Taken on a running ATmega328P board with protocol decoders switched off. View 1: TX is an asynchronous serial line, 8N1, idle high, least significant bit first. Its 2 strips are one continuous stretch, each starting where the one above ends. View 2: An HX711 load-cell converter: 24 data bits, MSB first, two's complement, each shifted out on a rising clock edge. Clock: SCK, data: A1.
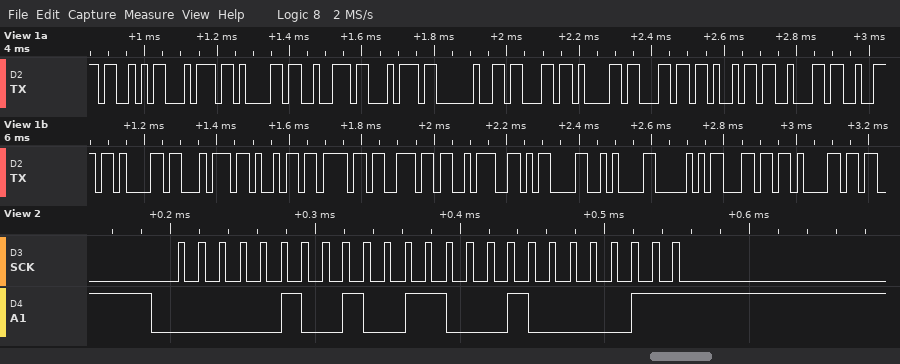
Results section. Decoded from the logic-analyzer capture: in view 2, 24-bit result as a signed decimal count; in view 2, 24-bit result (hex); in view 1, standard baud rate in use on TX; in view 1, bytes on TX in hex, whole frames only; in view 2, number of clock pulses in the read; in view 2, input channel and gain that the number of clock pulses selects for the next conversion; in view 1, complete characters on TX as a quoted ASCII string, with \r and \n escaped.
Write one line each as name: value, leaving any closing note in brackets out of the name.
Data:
in view 2, 24-bit result as a signed decimal count: 301187
in view 2, 24-bit result: 0x049883
in view 1, standard baud rate in use on TX: 57600 baud
in view 1, bytes on TX in hex, whole frames only: 53 74 61 72 74 20 63 61 6C 69 62 72 61 74 69 6F 6E 3A 0D 0A 50 6C 61
in view 2, number of clock pulses in the read: 25
in view 2, input channel and gain that the number of clock pulses selects for the next conversion: channel A, gain 128
in view 1, complete characters on TX as a quoted ASCII string, with \r and \n escaped: "Start calibration:\r\nPla"
